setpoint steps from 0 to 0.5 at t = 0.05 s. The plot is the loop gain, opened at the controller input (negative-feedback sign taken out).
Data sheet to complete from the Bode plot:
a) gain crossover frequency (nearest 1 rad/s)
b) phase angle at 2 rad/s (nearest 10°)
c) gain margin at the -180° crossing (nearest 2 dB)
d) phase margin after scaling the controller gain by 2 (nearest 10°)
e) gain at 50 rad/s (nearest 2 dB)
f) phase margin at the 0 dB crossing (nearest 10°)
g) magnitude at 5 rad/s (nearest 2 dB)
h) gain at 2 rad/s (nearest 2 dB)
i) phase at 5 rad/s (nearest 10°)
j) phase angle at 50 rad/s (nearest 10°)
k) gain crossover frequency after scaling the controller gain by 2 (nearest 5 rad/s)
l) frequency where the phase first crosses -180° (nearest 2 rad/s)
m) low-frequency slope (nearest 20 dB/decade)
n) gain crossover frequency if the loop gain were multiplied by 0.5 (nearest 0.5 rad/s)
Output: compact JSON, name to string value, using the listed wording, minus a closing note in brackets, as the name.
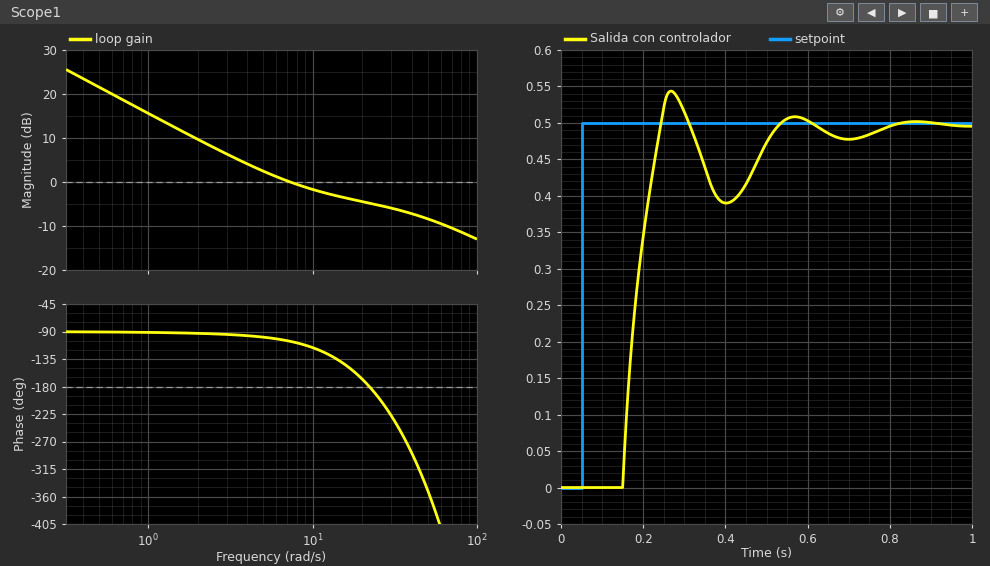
{"gain crossover frequency": "7 rad/s", "phase angle at 2 rad/s": "-90°", "gain margin at the -180° crossing": "4 dB", "phase margin after scaling the controller gain by 2": "-50°", "gain at 50 rad/s": "-8 dB", "phase margin at the 0 dB crossing": "70°", "magnitude at 5 rad/s": "2 dB", "gain at 2 rad/s": "10 dB", "phase at 5 rad/s": "-100°", "phase angle at 50 rad/s": "-350°", "gain crossover frequency after scaling the controller gain by 2": "30 rad/s", "frequency where the phase first crosses -180°": "22 rad/s", "low-frequency slope": "-20 dB/decade", "gain crossover frequency if the loop gain were multiplied by 0.5": "3.0 rad/s"}
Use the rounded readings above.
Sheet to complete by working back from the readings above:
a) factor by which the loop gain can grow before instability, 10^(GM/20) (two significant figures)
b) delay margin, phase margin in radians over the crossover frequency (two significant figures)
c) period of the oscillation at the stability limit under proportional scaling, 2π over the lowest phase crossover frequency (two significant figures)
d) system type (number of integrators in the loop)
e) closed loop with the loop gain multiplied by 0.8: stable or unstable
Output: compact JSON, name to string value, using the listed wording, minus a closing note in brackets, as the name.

{"factor by which the loop gain can grow before instability, 10^(GM/20)": "1.6", "delay margin, phase margin in radians over the crossover frequency": "0.17 s", "period of the oscillation at the stability limit under proportional scaling, 2π over the lowest phase crossover frequency": "0.29 s", "system type": "1", "closed loop with the loop gain multiplied by 0.8: stable or unstable": "stable"}
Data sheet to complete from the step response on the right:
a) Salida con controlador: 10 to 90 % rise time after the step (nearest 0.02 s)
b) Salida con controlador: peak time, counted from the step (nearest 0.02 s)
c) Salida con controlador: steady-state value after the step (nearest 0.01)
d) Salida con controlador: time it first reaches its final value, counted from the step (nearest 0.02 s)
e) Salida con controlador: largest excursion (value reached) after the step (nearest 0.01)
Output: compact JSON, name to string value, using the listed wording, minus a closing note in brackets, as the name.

{"Salida con controlador: 10 to 90 % rise time after the step": "0.08 s", "Salida con controlador: peak time, counted from the step": "0.22 s", "Salida con controlador: steady-state value after the step": "0.50", "Salida con controlador: time it first reaches its final value, counted from the step": "0.20 s", "Salida con controlador: largest excursion (value reached) after the step": "0.54"}
